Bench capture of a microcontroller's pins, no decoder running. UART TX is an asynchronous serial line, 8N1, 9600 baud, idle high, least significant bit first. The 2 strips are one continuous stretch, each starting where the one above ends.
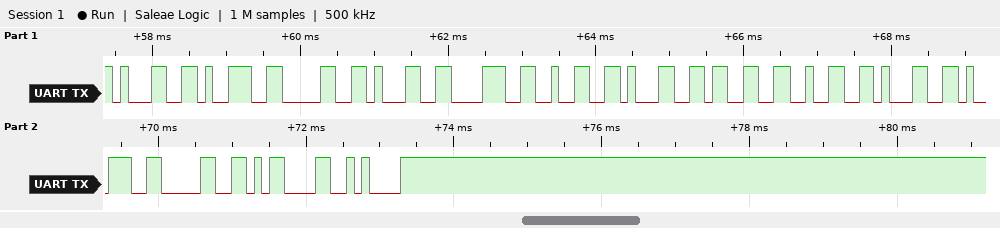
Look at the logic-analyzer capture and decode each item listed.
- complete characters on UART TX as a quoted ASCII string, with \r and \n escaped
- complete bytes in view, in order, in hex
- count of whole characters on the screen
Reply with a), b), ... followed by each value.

a) "190182132190\r\n"
b) 0x31 0x39 0x30 0x31 0x38 0x32 0x31 0x33 0x32 0x31 0x39 0x30 0x0D 0x0A
c) 14
